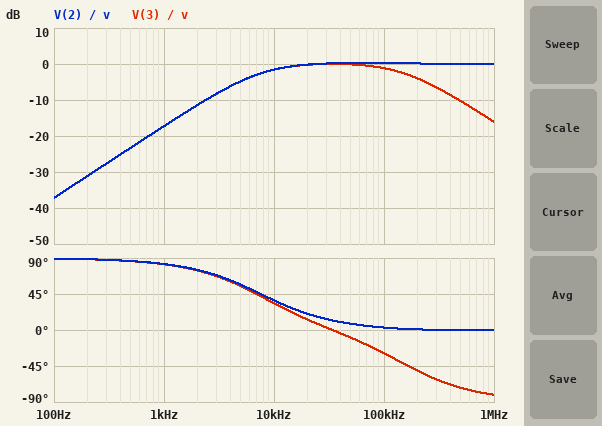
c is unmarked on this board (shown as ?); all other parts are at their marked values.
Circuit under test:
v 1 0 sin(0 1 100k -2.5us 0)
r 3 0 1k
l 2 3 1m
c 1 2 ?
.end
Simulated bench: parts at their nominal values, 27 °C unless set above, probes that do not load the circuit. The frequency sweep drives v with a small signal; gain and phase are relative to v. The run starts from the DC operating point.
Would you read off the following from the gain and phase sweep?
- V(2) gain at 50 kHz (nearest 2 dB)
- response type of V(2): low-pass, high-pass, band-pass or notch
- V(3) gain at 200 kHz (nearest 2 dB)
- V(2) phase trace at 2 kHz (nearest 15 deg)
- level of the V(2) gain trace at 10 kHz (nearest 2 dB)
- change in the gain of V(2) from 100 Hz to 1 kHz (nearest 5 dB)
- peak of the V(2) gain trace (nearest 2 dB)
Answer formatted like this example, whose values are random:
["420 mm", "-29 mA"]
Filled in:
["0 dB", "high-pass", "-4 dB", "75 deg", "-2 dB", "20 dB", "0 dB"]
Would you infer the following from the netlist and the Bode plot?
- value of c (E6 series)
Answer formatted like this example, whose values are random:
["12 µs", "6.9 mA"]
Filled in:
["22 nF"]
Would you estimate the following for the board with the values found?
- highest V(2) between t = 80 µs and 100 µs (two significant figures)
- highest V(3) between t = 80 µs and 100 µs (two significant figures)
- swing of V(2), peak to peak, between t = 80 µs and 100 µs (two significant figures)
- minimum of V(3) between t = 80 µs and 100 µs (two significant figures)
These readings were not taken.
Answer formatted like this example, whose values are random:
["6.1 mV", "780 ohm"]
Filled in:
["1.0 V", "860 mV", "2.1 V", "-890 mV"]
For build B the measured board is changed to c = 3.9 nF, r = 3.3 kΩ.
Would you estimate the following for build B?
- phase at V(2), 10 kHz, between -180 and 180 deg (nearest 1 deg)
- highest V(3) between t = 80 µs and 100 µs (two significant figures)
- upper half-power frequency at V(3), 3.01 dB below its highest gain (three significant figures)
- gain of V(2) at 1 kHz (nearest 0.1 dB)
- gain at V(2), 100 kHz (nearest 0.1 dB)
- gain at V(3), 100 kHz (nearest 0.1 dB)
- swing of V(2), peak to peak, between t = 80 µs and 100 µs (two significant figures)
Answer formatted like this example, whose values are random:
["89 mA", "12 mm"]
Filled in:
["52 deg", "1.0 V", "537 kHz", "-21.9 dB", "0.1 dB", "0 dB", "2.0 V"]
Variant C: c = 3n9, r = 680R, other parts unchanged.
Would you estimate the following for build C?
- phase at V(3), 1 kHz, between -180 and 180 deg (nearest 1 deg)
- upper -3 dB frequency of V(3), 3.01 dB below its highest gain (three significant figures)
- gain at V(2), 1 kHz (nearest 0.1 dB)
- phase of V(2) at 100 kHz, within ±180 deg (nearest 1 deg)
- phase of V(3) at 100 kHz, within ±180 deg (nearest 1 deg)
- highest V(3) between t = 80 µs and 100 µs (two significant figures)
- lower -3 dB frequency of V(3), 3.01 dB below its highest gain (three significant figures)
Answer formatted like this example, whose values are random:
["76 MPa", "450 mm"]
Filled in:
["89 deg", "151 kHz", "-35.6 dB", "25 deg", "-18 deg", "950 mV", "43.0 kHz"]
